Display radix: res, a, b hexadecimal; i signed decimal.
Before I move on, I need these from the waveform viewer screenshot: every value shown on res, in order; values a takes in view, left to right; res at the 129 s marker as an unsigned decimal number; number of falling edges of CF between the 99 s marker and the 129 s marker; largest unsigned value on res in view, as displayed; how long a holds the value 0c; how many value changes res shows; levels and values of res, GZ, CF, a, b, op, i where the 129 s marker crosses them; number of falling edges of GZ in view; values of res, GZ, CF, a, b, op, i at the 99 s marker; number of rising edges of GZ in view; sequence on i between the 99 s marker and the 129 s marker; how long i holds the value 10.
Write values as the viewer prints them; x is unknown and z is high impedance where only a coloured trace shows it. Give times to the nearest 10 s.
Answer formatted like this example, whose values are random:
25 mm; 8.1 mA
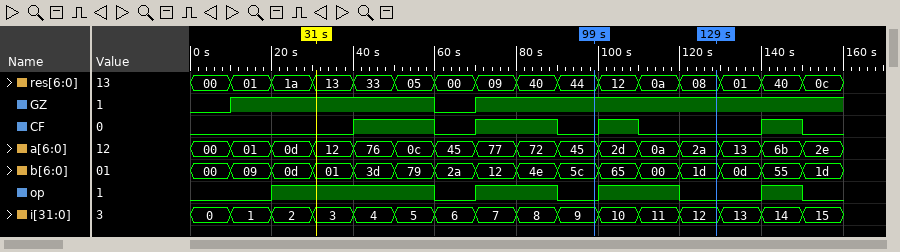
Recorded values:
00, 01, 1a, 13, 33, 05, 00, 09, 40, 44, 12, 0a, 08, 01, 40, 0c; 00, 01, 0d, 12, 76, 0c, 45, 77, 72, 45, 2d, 0a, 2a, 13, 6b, 2e; 8; 1; 44; 10 s; 15; res=08, GZ=1, CF=0, a=2a, b=1d, op=0, i=12; 1; res=44, GZ=1, CF=0, a=45, b=5c, op=0, i=9; 2; 9, 10, 11, 12; 10 s
